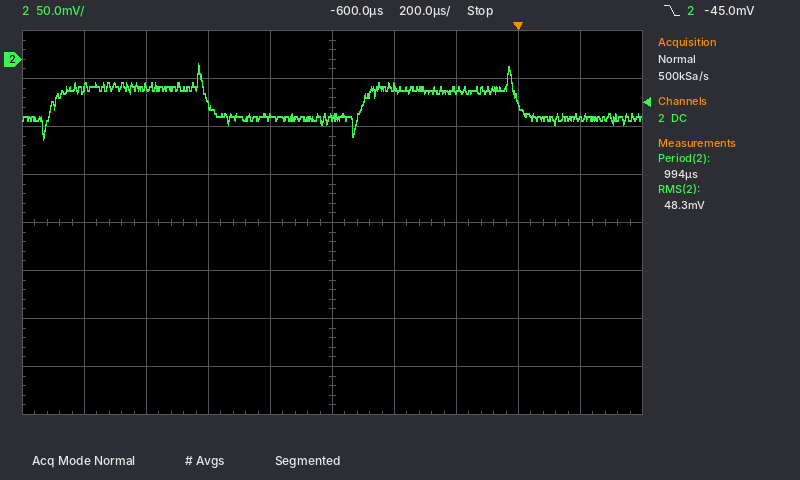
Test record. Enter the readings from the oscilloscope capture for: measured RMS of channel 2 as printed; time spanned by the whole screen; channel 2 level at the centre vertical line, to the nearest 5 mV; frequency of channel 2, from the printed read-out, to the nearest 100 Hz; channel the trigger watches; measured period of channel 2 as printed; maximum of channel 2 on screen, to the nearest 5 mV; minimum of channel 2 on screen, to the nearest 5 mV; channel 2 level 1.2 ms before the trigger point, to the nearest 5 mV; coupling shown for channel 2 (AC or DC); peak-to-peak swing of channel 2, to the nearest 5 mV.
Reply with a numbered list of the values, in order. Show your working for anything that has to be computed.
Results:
1. 48.3 mV
2. 2 ms
3. -60 mV
4. 1 / 994 µs ≈ 1.0 kHz
5. channel 2
6. 994 µs
7. -5 mV
8. -85 mV
9. -30 mV
10. DC
11. -5 mV − (-85 mV) = 80 mV
